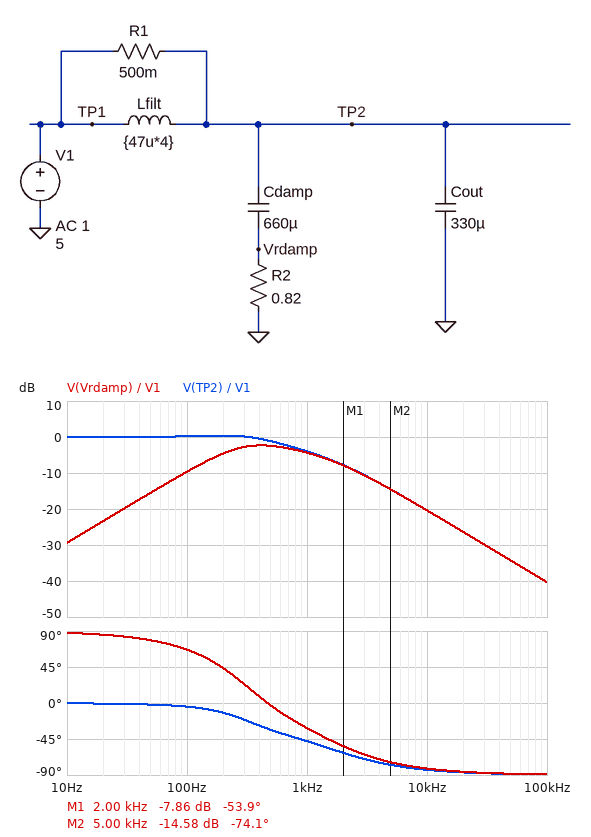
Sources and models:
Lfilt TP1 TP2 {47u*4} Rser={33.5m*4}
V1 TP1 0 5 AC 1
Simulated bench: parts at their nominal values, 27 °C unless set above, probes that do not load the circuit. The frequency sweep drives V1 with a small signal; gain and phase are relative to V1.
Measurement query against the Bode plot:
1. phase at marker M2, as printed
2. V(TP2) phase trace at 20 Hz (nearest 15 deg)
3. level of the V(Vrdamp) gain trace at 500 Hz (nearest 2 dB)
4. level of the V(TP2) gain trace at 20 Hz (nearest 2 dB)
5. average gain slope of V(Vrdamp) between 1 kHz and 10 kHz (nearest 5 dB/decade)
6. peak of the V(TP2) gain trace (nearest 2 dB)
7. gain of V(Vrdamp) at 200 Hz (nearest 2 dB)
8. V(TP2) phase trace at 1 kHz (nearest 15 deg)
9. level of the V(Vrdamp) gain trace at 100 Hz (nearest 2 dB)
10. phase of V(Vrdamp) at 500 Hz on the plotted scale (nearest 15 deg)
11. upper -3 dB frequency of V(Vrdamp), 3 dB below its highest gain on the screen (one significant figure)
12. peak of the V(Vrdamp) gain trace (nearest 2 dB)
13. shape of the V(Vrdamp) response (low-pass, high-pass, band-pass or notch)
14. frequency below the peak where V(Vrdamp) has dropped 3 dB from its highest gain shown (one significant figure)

-74.1 deg
0 deg
-2 dB
0 dB
-15 dB/decade
0 dB
-4 dB
-45 deg
-10 dB
0 deg
1 kHz
-2 dB
band-pass
200 Hz
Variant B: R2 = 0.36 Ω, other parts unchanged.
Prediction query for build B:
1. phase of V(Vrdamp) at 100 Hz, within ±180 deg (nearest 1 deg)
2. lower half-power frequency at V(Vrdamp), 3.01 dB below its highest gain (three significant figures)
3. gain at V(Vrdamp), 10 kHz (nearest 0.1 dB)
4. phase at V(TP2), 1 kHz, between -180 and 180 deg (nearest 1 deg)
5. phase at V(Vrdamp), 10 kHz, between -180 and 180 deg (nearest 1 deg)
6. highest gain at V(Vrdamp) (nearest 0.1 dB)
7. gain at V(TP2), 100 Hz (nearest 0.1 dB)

77 deg
227 Hz
-20.6 dB
-54 deg
-76 deg
-5.9 dB
0.3 dB
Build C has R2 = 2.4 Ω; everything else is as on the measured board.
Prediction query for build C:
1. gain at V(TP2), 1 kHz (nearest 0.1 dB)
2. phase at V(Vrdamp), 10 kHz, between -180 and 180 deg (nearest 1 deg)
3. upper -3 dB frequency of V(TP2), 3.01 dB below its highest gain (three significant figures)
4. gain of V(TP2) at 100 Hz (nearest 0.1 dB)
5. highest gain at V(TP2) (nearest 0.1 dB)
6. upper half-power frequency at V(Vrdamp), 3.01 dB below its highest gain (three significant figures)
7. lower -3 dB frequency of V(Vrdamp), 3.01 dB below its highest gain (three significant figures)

-1.9 dB
-85 deg
1.15 kHz
0 dB
0.3 dB
1.19 kHz
100 Hz
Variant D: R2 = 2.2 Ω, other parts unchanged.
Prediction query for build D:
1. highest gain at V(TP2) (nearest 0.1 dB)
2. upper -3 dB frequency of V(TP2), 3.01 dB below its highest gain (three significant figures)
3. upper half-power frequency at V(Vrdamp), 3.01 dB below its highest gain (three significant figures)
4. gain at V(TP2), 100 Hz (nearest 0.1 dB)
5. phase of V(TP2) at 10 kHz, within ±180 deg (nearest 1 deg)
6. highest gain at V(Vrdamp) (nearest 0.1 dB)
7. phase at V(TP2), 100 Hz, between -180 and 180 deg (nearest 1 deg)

0.2 dB
1.14 kHz
1.20 kHz
0 dB
-86 deg
-0.1 dB
-4 deg
